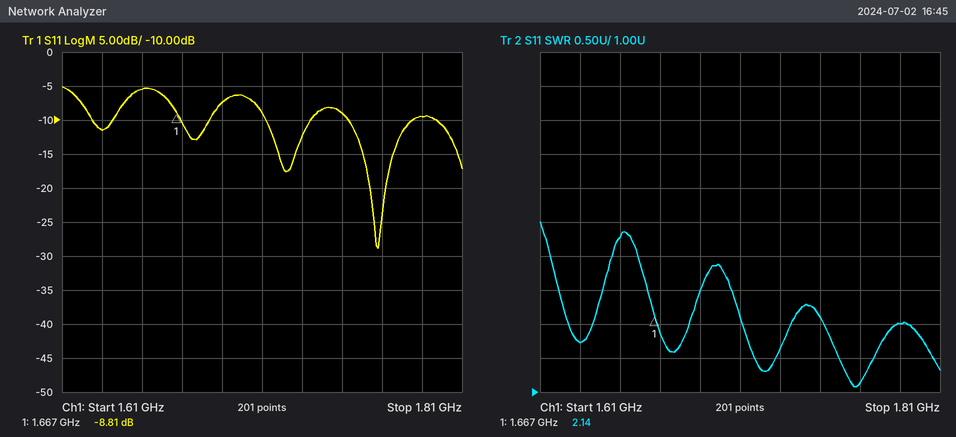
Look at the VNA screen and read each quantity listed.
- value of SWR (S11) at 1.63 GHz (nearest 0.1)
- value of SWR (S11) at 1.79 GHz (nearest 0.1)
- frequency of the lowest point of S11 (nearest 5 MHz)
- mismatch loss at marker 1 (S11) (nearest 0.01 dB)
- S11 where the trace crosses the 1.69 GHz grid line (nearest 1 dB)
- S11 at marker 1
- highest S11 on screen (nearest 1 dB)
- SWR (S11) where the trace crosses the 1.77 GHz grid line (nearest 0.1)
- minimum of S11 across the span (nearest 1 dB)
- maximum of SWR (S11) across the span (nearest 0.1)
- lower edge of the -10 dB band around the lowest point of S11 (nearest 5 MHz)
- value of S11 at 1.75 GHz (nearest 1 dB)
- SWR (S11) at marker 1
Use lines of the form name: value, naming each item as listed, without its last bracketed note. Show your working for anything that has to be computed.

value of SWR (S11) at 1.63 GHz: 1.7
value of SWR (S11) at 1.79 GHz: 2.0
frequency of the lowest point of S11: 1.770 GHz
mismatch loss at marker 1 (S11): −10 log10(1 − 10^(-8.81/10)) ≈ 0.61 dB
S11 where the trace crosses the 1.69 GHz grid line: -7 dB
S11 at marker 1: -8.81 dB
highest S11 on screen: -5 dB
SWR (S11) where the trace crosses the 1.77 GHz grid line: 1.1
minimum of S11 across the span: -29 dB
maximum of SWR (S11) across the span: 3.5
lower edge of the -10 dB band around the lowest point of S11: 1.755 GHz
value of S11 at 1.75 GHz: -9 dB
SWR (S11) at marker 1: 2.14
